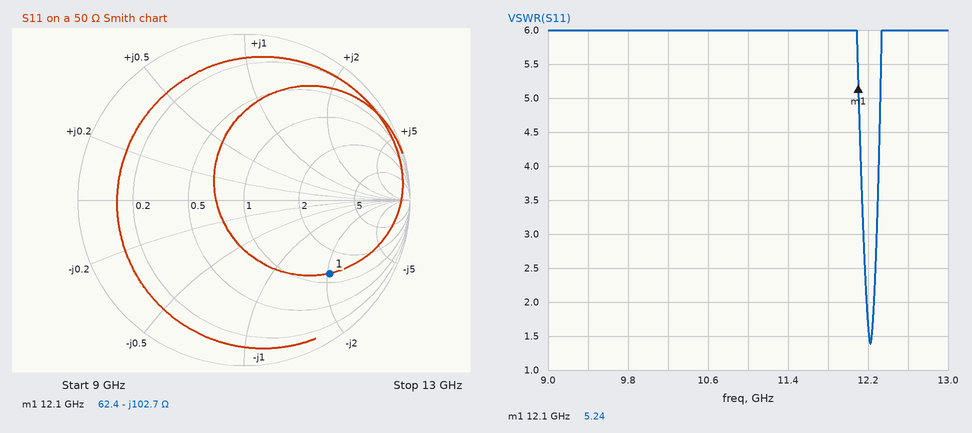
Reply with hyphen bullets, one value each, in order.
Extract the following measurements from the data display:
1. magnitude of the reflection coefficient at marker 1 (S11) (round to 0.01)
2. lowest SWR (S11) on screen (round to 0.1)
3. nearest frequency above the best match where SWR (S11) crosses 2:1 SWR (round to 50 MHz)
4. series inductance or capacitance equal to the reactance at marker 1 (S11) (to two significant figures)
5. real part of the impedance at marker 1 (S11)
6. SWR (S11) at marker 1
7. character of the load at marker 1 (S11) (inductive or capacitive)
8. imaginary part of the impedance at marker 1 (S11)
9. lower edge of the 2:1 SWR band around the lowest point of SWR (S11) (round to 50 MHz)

- 0.68
- 1.4
- 12.25 GHz
- 130 fF
- 62.4 Ω
- 5.24
- capacitive
- -102.7 Ω
- 12.20 GHz
